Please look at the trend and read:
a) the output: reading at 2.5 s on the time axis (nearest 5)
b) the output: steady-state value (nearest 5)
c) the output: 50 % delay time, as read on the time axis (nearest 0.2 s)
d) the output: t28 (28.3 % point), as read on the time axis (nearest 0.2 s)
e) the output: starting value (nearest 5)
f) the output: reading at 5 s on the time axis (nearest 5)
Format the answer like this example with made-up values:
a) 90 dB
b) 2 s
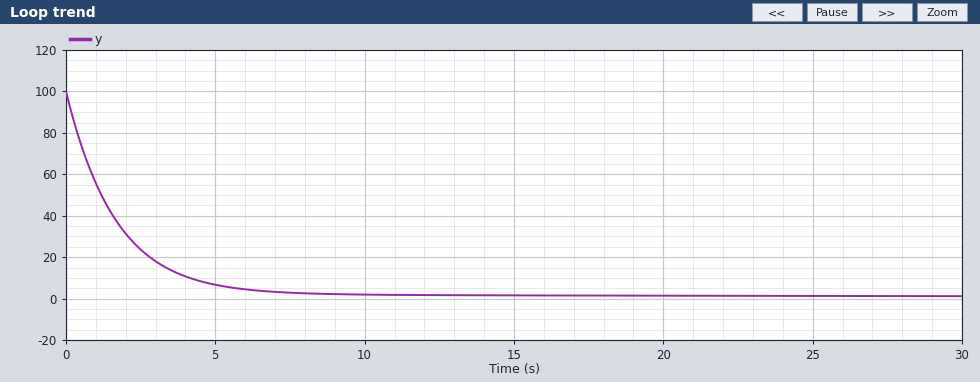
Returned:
a) 25
b) 0
c) 1.2 s
d) 0.6 s
e) 100
f) 5
